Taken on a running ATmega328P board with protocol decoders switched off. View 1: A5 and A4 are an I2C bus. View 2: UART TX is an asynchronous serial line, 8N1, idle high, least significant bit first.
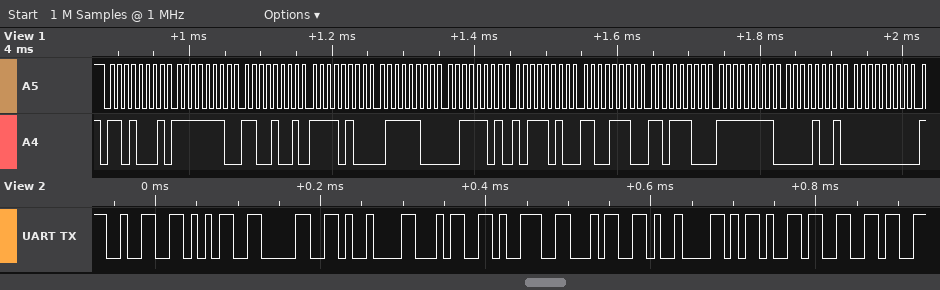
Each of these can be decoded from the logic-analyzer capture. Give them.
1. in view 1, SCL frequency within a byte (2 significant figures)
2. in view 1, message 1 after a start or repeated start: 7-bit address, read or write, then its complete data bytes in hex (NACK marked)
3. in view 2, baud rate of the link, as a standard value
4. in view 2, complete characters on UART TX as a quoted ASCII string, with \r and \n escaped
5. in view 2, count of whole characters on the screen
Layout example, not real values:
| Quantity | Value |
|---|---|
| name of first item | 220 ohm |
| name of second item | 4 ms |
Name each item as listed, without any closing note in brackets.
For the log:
| Quantity | Value |
|---|---|
| in view 1, SCL frequency within a byte | 100 kHz |
| in view 1, message 1 after a start or repeated start: 7-bit address, read or write, then its complete data bytes in hex | 0x68 read: FE C9 F4 7C 3D BA CE DC FF 09 00 |
| in view 2, baud rate of the link, as a standard value | 115200 baud |
| in view 2, complete characters on UART TX as a quoted ASCII string, with \r and \n escaped | "250\t494\t-3" |
| in view 2, count of whole characters on the screen | 10 |
